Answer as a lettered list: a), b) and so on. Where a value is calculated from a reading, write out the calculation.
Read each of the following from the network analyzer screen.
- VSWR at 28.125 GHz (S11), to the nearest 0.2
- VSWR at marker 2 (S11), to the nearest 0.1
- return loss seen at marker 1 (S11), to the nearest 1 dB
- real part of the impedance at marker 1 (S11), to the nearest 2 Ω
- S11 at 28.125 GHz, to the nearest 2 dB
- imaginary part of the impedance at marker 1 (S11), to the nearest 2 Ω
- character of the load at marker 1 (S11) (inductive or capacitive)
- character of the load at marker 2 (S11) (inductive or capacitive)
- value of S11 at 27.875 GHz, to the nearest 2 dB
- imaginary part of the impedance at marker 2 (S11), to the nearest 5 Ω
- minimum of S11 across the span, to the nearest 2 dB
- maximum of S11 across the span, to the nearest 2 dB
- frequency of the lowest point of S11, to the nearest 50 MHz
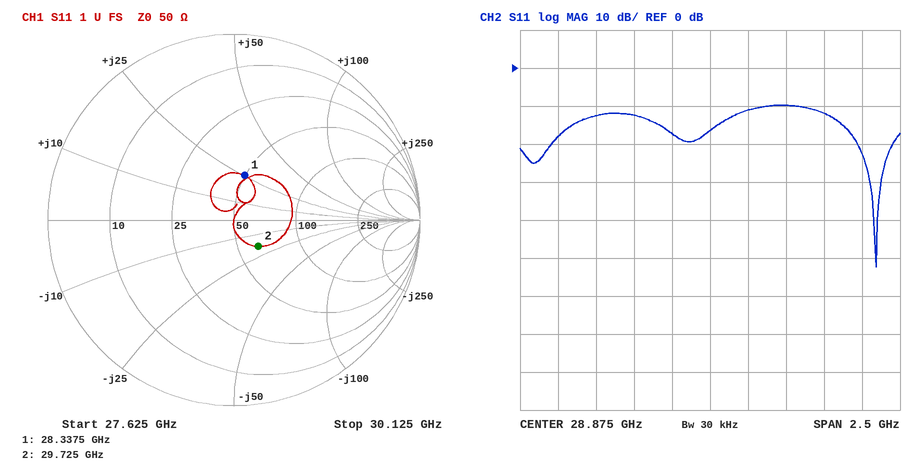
a) |Γ| = 10^(-12/20) = 0.2512; VSWR = (1 + 0.2512)/(1 − 0.2512) ≈ 1.67, so 1.6 to the nearest 0.2
b) 1.5
c) 12 dB
d) 50 Ω
e) -12 dB
f) +26 Ω
g) inductive
h) capacitive
i) -18 dB
j) -20 Ω
k) -52 dB
l) -10 dB
m) 29.95 GHz
